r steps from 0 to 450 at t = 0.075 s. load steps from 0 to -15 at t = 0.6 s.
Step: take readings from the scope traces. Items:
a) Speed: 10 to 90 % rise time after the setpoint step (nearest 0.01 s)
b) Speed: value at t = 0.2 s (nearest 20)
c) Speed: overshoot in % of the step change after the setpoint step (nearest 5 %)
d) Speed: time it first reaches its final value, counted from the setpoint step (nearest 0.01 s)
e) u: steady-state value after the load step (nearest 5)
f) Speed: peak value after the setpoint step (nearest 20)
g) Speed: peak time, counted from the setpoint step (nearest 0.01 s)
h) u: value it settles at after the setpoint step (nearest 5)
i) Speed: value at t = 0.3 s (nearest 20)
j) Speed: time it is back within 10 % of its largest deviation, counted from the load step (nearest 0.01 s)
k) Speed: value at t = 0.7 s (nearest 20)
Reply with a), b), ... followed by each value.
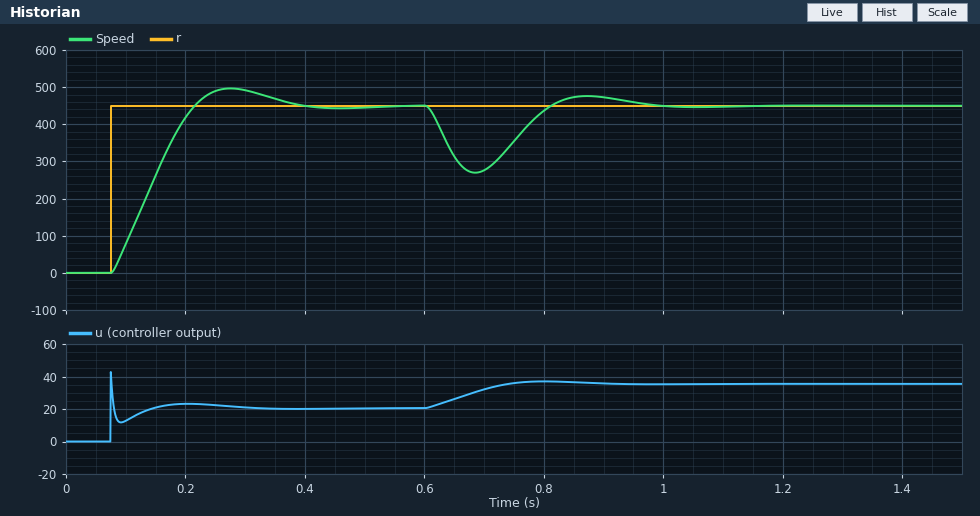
a) 0.10 s
b) 420
c) 10 %
d) 0.14 s
e) 35
f) 500
g) 0.20 s
h) 20
i) 500
j) 0.32 s
k) 280
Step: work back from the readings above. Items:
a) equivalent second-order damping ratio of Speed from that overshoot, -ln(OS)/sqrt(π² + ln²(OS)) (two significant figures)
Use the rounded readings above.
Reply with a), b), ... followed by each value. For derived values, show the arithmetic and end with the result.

a) ln(0.1) = -2.303; 2.303 / sqrt(9.870 + 5.302) = 0.59
